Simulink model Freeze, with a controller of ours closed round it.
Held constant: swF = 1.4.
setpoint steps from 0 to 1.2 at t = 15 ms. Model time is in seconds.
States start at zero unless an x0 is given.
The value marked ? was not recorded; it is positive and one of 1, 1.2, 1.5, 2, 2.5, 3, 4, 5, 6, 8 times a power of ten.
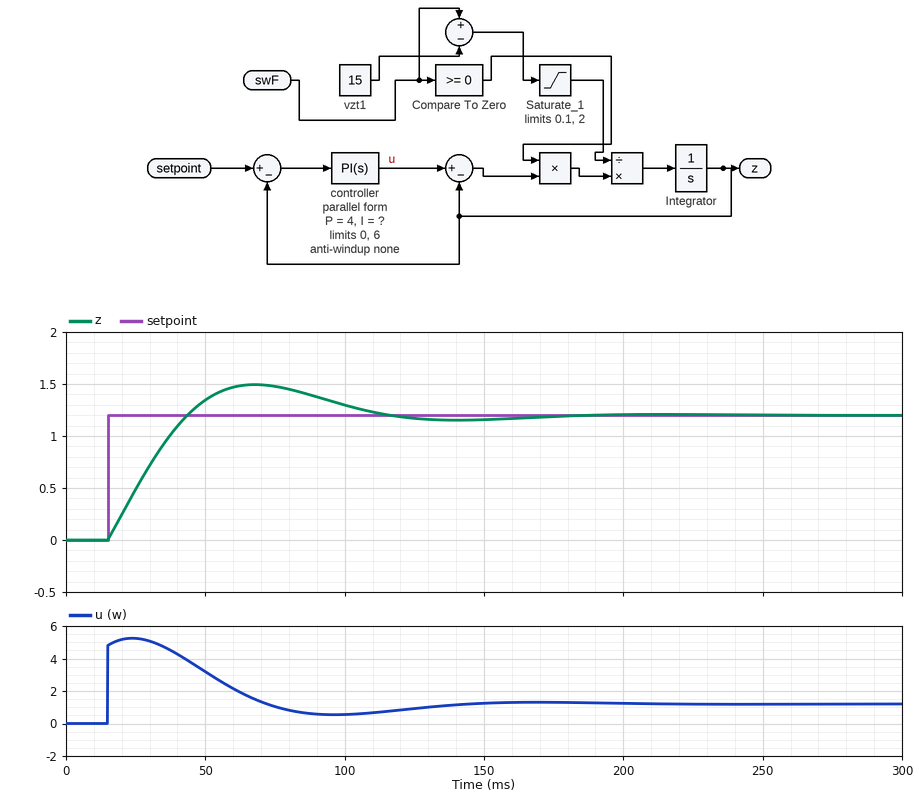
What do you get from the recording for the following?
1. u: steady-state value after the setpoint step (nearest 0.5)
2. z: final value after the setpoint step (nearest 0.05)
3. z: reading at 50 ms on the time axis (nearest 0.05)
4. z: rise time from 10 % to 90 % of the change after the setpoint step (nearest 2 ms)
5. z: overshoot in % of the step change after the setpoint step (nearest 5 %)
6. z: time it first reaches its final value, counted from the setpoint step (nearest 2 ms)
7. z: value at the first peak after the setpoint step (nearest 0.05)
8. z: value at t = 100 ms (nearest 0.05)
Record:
1.0
1.20
1.35
22 ms
25 %
28 ms
1.50
1.30
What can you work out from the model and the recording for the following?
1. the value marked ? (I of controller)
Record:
250
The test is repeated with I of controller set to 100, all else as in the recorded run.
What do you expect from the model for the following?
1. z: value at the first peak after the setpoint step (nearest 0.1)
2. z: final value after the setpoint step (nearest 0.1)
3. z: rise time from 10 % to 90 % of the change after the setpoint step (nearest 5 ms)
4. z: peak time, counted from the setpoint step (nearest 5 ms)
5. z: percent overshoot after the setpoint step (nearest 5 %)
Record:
1.3
1.2
35 ms
80 ms
10 %
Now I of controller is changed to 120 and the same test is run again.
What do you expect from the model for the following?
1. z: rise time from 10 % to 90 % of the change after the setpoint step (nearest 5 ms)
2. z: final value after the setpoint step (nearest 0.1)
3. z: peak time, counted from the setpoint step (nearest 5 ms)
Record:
30 ms
1.2
75 ms
